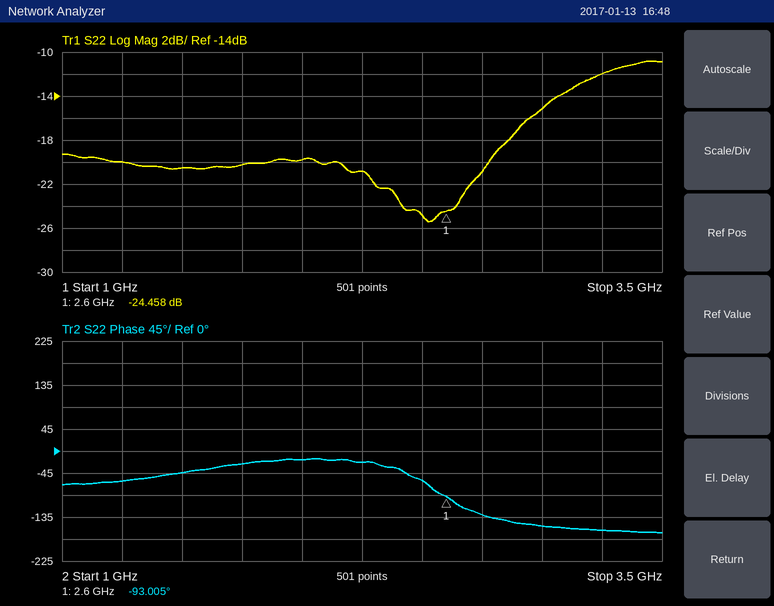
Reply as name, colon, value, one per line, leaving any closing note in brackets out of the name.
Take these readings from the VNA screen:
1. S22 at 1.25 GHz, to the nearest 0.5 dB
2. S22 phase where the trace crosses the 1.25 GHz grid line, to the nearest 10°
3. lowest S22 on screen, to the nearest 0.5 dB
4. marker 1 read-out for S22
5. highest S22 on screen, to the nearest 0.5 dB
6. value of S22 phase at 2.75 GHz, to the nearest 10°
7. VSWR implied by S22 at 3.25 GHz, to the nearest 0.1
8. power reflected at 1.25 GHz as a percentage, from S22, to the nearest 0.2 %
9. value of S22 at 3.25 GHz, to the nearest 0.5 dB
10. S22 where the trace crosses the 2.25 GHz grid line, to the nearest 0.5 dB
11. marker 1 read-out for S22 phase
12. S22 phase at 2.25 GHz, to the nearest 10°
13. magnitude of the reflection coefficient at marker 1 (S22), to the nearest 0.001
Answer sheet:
S22 at 1.25 GHz, to the nearest 0.5 dB: -20.0 dB
S22 phase where the trace crosses the 1.25 GHz grid line, to the nearest 10°: -60°
lowest S22 on screen, to the nearest 0.5 dB: -25.5 dB
marker 1 read-out for S22: -24.458 dB
highest S22 on screen, to the nearest 0.5 dB: -11.0 dB
value of S22 phase at 2.75 GHz, to the nearest 10°: -130°
VSWR implied by S22 at 3.25 GHz, to the nearest 0.1: 1.7
power reflected at 1.25 GHz as a percentage, from S22, to the nearest 0.2 %: 1.0 %
value of S22 at 3.25 GHz, to the nearest 0.5 dB: -12.0 dB
S22 where the trace crosses the 2.25 GHz grid line, to the nearest 0.5 dB: -21.0 dB
marker 1 read-out for S22 phase: -93.005°
S22 phase at 2.25 GHz, to the nearest 10°: -20°
magnitude of the reflection coefficient at marker 1 (S22), to the nearest 0.001: 0.060
